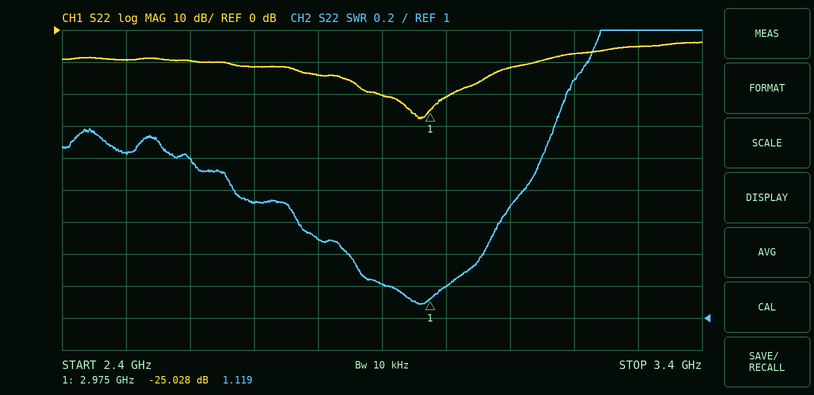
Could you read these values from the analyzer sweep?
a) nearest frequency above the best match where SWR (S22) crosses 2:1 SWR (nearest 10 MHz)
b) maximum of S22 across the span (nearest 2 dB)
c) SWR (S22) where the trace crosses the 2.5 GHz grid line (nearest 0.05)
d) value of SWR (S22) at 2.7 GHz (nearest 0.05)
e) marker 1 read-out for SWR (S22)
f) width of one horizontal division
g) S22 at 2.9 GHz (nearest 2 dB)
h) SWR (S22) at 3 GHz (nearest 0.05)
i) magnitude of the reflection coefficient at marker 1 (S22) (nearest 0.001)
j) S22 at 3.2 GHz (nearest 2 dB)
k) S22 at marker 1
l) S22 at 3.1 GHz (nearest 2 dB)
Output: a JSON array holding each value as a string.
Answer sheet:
["3.15 GHz", "-4 dB", "2.05", "1.70", "1.119", "100 MHz", "-20 dB", "1.20", "0.056", "-8 dB", "-25.028 dB", "-12 dB"]
